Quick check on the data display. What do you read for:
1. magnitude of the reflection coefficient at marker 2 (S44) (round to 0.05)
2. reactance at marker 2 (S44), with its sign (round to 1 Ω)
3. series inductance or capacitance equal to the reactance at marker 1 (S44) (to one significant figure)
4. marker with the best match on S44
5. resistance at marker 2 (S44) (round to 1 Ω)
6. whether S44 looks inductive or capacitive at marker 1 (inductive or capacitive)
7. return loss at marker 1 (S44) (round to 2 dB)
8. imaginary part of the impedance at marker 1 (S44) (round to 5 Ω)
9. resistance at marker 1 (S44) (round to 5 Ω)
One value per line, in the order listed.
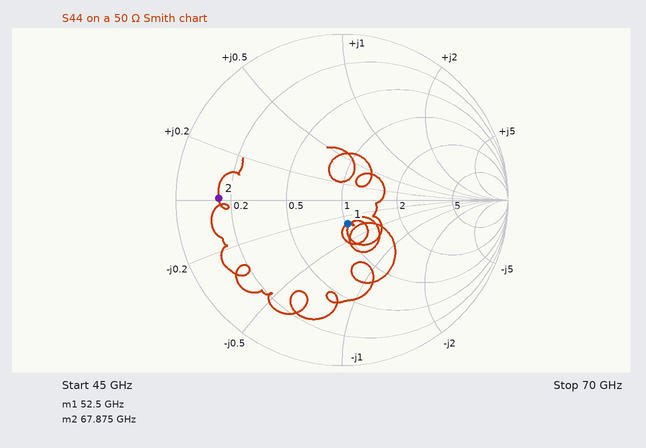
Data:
0.75
0 Ω
200 fF
marker 1
7 Ω
capacitive
16 dB
-15 Ω
50 Ω
